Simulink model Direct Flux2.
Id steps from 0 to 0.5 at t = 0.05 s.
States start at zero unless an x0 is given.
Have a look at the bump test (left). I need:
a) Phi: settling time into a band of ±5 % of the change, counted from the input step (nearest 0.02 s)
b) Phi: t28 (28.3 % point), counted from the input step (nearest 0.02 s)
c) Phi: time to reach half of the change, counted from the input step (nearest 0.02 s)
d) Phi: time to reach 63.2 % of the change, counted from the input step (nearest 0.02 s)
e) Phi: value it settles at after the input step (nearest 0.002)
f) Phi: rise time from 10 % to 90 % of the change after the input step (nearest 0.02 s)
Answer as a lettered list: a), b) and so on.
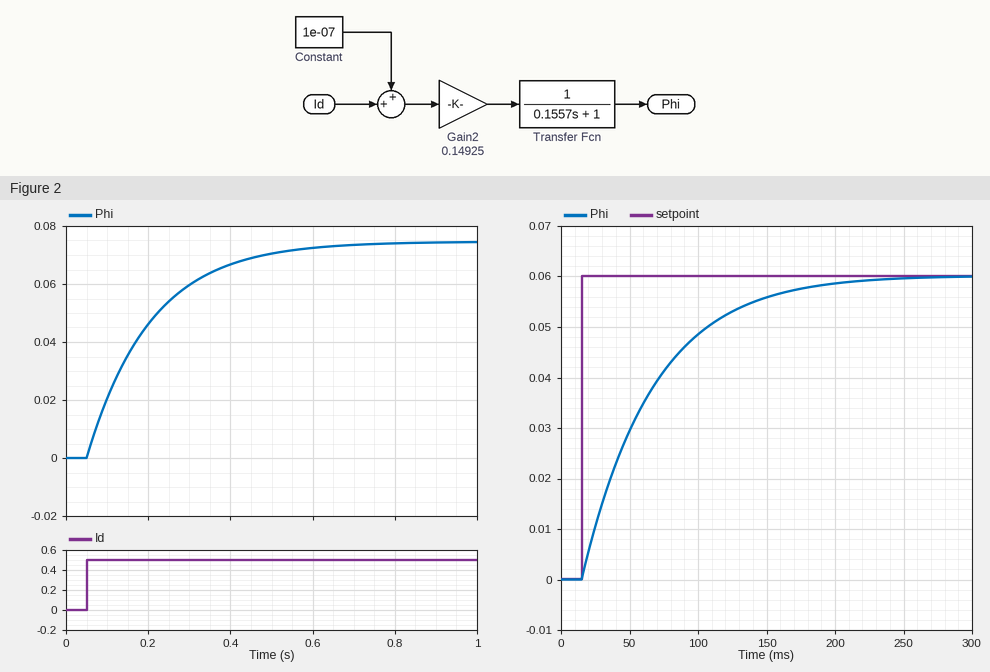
a) 0.46 s
b) 0.06 s
c) 0.10 s
d) 0.16 s
e) 0.074
f) 0.34 s
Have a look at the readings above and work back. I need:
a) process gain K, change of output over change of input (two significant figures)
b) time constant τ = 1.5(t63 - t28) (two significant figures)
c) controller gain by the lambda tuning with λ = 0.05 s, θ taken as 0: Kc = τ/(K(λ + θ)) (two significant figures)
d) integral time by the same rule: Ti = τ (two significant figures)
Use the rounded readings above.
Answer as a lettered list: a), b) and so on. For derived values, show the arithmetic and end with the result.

a) (0.074 - 0) / 0.5 = 0.15
b) 1.5 × (0.16 - 0.06) = 0.15 s
c) 0.15 / (0.15 × (0.05 + 0)) = 20
d) 0.15 s
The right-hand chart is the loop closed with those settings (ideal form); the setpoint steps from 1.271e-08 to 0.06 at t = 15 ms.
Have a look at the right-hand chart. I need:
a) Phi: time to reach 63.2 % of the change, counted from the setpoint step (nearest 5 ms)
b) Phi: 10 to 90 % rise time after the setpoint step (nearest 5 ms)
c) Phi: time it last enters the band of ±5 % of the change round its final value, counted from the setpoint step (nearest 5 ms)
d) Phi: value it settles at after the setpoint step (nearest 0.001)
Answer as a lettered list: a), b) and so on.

a) 50 ms
b) 110 ms
c) 150 ms
d) 0.060
